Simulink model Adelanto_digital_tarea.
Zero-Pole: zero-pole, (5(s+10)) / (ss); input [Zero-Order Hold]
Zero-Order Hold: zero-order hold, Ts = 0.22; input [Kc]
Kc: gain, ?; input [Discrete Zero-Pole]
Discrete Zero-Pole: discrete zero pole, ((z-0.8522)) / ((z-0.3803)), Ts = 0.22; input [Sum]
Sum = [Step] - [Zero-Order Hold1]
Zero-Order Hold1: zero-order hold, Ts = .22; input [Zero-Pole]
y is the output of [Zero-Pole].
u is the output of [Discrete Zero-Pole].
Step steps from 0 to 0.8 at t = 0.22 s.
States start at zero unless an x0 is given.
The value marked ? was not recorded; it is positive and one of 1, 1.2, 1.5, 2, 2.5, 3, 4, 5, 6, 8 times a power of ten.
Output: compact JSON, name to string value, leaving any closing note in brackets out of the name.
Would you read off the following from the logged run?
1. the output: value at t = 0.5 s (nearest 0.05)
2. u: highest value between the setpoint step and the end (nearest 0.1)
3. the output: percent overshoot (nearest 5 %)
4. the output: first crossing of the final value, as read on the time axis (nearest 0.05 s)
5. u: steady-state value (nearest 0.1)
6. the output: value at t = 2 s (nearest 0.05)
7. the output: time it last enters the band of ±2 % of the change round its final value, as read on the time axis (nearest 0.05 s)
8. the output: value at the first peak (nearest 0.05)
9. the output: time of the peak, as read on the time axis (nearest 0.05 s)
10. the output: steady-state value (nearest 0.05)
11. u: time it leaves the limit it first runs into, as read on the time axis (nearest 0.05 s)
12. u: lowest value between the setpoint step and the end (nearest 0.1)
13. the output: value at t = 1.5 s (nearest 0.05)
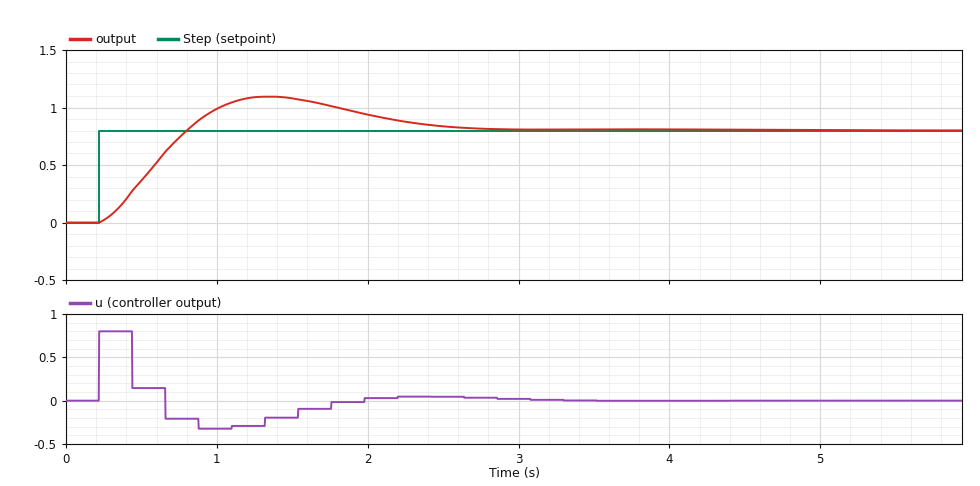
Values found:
{"the output: value at t = 0.5 s": "0.35", "u: highest value between the setpoint step and the end": "0.8", "the output: percent overshoot": "35 %", "the output: first crossing of the final value, as read on the time axis": "0.80 s", "u: steady-state value": "0.0", "the output: value at t = 2 s": "0.95", "the output: time it last enters the band of ±2 % of the change round its final value, as read on the time axis": "2.75 s", "the output: value at the first peak": "1.10", "the output: time of the peak, as read on the time axis": "1.35 s", "the output: steady-state value": "0.80", "u: time it leaves the limit it first runs into, as read on the time axis": "0.45 s", "u: lowest value between the setpoint step and the end": "-0.3", "the output: value at t = 1.5 s": "1.10"}
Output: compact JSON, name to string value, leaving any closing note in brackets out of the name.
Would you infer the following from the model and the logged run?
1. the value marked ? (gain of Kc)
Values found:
{"the value marked ?": "0.15"}
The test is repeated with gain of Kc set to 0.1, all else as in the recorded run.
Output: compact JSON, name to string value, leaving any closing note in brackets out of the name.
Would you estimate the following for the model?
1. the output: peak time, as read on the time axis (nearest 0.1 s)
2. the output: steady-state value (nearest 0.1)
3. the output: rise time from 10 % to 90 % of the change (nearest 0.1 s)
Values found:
{"the output: peak time, as read on the time axis": "1.8 s", "the output: steady-state value": "0.8", "the output: rise time from 10 % to 90 % of the change": "0.6 s"}
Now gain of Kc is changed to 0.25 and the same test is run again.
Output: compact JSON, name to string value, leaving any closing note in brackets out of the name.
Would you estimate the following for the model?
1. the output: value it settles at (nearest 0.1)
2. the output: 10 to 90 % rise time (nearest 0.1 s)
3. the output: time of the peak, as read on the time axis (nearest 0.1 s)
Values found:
{"the output: value it settles at": "0.8", "the output: 10 to 90 % rise time": "0.3 s", "the output: time of the peak, as read on the time axis": "1.0 s"}
